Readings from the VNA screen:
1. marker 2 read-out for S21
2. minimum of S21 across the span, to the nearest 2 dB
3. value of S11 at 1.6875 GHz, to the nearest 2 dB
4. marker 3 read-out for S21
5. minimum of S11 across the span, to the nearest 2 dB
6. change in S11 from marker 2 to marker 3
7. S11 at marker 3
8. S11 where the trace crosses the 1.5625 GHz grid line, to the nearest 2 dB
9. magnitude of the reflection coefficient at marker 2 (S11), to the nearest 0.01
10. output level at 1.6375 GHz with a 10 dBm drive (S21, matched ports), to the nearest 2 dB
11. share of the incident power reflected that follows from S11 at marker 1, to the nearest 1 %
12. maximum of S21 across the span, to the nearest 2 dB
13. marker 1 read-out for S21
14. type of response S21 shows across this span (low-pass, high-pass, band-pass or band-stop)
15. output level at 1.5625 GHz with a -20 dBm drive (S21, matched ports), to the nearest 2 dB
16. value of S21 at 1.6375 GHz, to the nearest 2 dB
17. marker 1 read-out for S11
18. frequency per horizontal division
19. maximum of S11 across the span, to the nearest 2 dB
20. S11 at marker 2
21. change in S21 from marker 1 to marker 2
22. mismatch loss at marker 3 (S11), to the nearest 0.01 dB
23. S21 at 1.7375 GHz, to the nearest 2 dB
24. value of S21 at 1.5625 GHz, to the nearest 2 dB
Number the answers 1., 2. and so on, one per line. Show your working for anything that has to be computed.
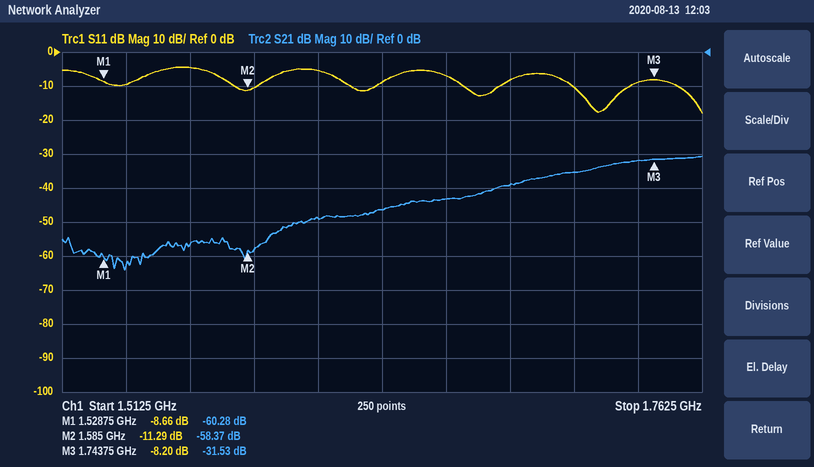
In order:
1. -58.37 dB
2. -64 dB
3. -8 dB
4. -31.53 dB
5. -18 dB
6. -8.2 − (-11.29) = 3.09 dB
7. -8.20 dB
8. -4 dB
9. 10^(-11.29/20) ≈ 0.27
10. 10 dBm + (-46 dB) = -36 dBm
11. 10^(-8.66/10) ≈ 14 %
12. -30 dB
13. -60.28 dB
14. high-pass
15. -20 dBm + (-56 dB) = -76 dBm
16. -46 dB
17. -8.66 dB
18. 25 MHz
19. -4 dB
20. -11.29 dB
21. -58.37 − (-60.28) = 1.91 dB
22. −10 log10(1 − 10^(-8.2/10)) ≈ 0.71 dB
23. -32 dB
24. -56 dB
